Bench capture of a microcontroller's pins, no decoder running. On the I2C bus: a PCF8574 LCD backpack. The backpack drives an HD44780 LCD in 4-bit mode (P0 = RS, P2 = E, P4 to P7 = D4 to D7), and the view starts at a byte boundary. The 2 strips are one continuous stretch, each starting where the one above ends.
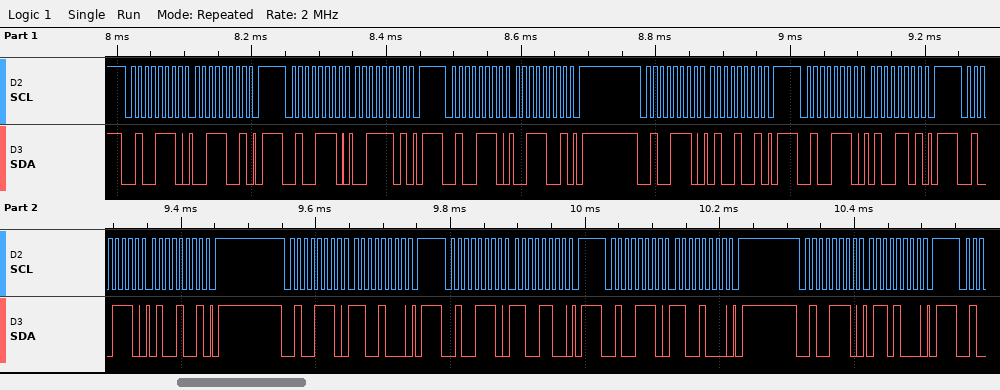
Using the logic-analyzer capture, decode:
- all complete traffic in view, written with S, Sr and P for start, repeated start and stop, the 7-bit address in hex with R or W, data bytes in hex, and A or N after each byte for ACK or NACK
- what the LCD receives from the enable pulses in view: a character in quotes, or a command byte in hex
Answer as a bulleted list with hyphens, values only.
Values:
- S 27W A 39 A P S 27W A 3D A P S 27W A 39 A P S 27W A 49 A P S 27W A 4D A P S 27W A 49 A P S 27W A C8 A P S 27W A CC A P S 27W A C8 A P S 27W A 68 A P
- '4'
